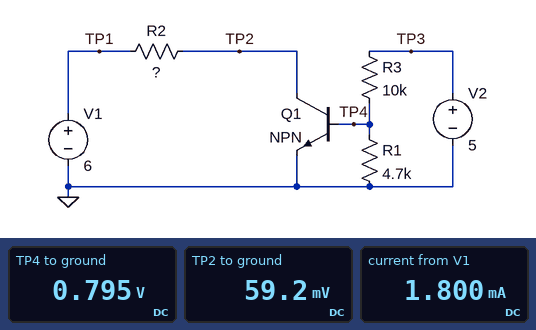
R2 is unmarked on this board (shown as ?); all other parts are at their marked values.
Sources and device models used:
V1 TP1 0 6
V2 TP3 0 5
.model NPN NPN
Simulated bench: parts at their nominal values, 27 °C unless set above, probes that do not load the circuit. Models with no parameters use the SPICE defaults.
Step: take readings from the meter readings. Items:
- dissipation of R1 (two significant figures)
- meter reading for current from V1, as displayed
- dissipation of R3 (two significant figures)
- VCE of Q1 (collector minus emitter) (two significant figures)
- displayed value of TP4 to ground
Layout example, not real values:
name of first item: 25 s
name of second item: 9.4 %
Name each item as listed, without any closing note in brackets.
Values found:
dissipation of R1: 130 µW
meter reading for current from V1, as displayed: 1.800 mA
dissipation of R3: 1.8 mW
VCE of Q1 (collector minus emitter): 59 mV
displayed value of TP4 to ground: 0.795 V
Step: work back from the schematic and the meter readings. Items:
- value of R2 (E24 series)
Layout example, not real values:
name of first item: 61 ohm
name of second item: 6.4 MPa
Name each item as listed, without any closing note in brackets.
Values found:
value of R2: 3.3 kΩ
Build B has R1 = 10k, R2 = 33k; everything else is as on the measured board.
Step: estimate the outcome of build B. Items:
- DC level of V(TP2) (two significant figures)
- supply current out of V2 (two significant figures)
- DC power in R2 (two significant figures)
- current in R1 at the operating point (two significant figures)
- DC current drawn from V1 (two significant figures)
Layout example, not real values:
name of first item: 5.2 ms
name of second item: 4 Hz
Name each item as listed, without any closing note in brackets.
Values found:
DC level of V(TP2): 24 mV
supply current out of V2: 420 µA
DC power in R2: 1.1 mW
current in R1 at the operating point: 77 µA
DC current drawn from V1: 180 µA
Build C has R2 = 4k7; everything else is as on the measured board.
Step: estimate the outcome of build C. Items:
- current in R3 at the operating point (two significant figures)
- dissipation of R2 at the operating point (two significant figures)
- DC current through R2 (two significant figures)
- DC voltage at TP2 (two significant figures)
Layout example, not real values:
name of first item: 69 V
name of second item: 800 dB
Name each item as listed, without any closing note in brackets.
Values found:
current in R3 at the operating point: 420 µA
dissipation of R2 at the operating point: 7.5 mW
DC current through R2: 1.3 mA
DC voltage at TP2: 52 mV
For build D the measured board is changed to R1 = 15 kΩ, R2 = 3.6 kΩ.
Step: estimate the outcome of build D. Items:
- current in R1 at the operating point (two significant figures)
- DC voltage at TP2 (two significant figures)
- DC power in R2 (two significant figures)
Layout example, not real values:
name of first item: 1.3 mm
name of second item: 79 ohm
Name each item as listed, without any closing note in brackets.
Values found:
current in R1 at the operating point: 53 µA
DC voltage at TP2: 50 mV
DC power in R2: 9.8 mW
